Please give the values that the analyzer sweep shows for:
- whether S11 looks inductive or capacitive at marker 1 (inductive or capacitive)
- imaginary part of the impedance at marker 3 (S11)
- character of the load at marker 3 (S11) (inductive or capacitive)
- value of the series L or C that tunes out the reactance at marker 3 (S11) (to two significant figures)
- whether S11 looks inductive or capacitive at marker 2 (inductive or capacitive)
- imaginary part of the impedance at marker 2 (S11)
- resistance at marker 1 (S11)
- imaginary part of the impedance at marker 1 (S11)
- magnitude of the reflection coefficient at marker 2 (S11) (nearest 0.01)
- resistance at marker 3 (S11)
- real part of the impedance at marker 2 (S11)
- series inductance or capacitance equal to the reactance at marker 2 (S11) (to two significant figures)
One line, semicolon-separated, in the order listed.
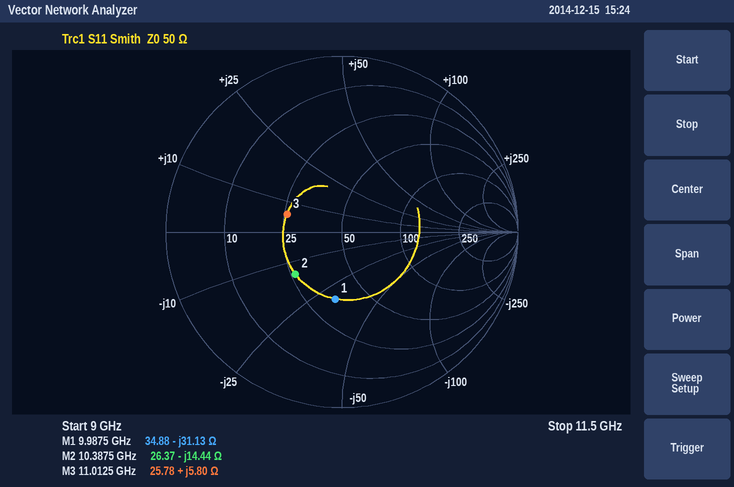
capacitive; +5.80 Ω; inductive; 2.5 pF; capacitive; -14.44 Ω; 34.88 Ω; -31.13 Ω; 0.36; 25.78 Ω; 26.37 Ω; 1.1 pF
